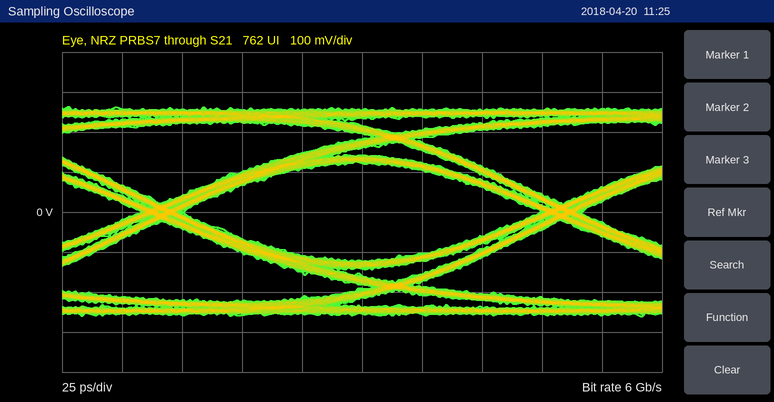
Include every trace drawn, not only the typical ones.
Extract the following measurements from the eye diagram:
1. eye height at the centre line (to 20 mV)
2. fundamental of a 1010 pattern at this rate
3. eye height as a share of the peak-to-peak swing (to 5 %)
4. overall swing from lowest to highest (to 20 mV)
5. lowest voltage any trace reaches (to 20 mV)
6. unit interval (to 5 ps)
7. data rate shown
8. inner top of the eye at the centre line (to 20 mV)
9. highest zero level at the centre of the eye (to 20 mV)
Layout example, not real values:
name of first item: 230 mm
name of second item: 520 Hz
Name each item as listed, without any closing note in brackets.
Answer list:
eye height at the centre line: 240 mV
fundamental of a 1010 pattern at this rate: 3 GHz
eye height as a share of the peak-to-peak swing: 45 %
overall swing from lowest to highest: 520 mV
lowest voltage any trace reaches: -260 mV
unit interval: 165 ps
data rate shown: 6 Gb/s
inner top of the eye at the centre line: 120 mV
highest zero level at the centre of the eye: -120 mV
